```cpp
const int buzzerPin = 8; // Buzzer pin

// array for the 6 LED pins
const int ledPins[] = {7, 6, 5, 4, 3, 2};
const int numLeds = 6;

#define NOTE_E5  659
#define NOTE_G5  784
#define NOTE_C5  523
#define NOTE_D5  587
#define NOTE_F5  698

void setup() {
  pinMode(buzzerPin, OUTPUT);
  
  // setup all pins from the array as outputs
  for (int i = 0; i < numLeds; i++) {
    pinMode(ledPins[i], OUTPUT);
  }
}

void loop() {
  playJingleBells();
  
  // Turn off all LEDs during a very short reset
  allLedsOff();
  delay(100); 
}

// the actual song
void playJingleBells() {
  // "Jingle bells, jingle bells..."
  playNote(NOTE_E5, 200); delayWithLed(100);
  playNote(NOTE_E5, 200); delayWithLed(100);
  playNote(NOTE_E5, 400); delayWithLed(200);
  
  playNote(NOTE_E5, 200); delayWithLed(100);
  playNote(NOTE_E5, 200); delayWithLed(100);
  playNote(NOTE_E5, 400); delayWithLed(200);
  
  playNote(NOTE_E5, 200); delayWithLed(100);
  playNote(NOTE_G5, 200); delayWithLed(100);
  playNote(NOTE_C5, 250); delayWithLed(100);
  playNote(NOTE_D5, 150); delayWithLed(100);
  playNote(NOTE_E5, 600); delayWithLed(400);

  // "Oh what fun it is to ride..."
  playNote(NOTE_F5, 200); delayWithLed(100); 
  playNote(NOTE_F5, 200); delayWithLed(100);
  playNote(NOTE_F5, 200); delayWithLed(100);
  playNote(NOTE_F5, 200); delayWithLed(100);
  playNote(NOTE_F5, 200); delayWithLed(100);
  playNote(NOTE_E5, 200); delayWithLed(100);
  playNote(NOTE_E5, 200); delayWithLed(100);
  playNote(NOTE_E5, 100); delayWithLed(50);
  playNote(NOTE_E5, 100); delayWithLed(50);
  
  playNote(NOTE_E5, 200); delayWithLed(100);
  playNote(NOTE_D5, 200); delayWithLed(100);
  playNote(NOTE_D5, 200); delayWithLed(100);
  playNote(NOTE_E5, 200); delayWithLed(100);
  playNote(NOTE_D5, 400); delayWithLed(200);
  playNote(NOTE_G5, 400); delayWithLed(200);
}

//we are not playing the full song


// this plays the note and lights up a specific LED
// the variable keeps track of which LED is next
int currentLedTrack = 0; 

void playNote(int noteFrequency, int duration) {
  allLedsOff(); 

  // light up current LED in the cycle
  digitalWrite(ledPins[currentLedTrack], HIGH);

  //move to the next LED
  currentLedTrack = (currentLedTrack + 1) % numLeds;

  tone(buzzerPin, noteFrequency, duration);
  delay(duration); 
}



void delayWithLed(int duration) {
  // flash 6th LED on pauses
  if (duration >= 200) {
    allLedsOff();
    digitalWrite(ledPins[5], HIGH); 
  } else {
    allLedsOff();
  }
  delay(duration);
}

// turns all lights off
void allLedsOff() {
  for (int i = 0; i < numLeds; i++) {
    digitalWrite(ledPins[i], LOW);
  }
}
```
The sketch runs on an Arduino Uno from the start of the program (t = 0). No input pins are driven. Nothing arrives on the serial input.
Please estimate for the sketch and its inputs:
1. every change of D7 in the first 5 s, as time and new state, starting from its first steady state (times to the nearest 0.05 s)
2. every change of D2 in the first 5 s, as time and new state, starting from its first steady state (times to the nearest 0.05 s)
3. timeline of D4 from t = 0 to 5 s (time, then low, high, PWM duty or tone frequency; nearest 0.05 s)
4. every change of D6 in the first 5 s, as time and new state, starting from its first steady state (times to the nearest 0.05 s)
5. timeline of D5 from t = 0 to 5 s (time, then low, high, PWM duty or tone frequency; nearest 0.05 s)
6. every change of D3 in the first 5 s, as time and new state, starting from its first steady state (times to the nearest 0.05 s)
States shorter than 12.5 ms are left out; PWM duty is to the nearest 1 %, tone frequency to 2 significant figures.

0 s high; 0.2 s low; 2.4 s high; 2.6 s low; 4.9 s high
0 s low; 1 s high; 1.2 s low; 1.8 s high; 2.4 s low; 4.2 s high; 4.8 s low
0 s low; 1.2 s high; 1.4 s low; 3.35 s high; 3.5 s low
0 s low; 0.3 s high; 0.5 s low; 2.7 s high; 2.9 s low
0 s low; 0.6 s high; 1 s low; 3 s high; 3.25 s low
0 s low; 1.5 s high; 1.7 s low; 3.6 s high; 4.2 s low
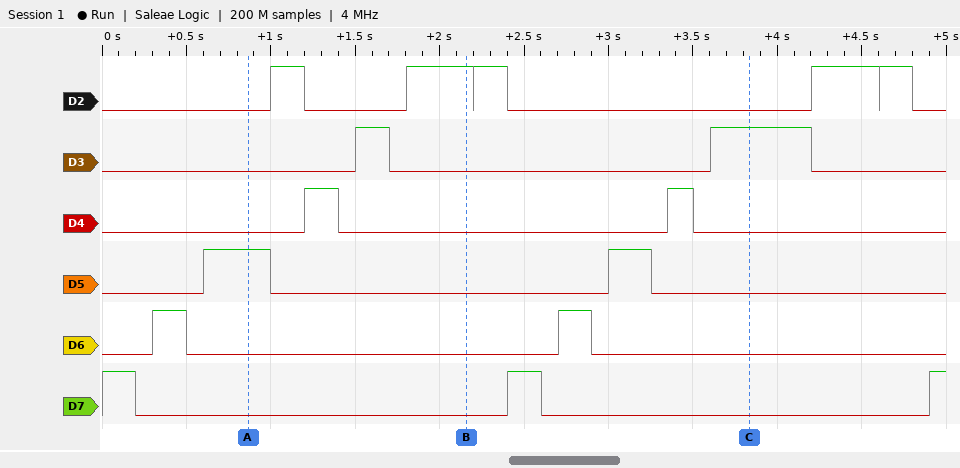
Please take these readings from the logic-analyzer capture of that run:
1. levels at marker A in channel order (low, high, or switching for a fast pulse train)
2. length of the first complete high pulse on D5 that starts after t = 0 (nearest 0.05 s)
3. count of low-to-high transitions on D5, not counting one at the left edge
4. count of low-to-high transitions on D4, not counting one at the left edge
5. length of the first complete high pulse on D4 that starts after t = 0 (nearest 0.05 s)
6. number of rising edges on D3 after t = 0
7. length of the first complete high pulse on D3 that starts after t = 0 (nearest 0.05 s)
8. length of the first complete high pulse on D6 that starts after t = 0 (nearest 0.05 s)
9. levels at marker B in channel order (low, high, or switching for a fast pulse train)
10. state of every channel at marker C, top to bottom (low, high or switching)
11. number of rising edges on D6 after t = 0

D2 low, D3 low, D4 low, D5 high, D6 low, D7 low
0.40 s
2
2
0.20 s
2
0.20 s
0.20 s
D2 high, D3 low, D4 low, D5 low, D6 low, D7 low
D2 low, D3 high, D4 low, D5 low, D6 low, D7 low
2
